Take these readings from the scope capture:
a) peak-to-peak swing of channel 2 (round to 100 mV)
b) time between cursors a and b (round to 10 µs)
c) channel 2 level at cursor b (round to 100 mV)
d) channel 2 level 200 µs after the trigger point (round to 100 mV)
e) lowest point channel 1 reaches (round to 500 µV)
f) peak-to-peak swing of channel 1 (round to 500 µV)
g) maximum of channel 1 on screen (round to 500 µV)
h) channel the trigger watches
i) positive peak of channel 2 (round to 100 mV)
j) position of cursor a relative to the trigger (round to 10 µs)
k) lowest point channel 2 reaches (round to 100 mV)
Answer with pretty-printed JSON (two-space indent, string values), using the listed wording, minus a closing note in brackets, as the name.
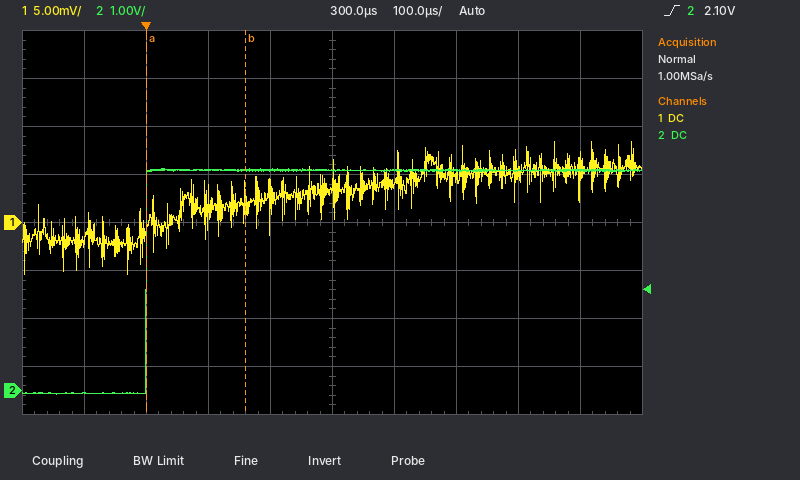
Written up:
{
  "peak-to-peak swing of channel 2": "4.7 V",
  "time between cursors a and b": "160 µs",
  "channel 2 level at cursor b": "4.6 V",
  "channel 2 level 200 µs after the trigger point": "4.6 V",
  "lowest point channel 1 reaches": "-5.5 mV",
  "peak-to-peak swing of channel 1": "14.0 mV",
  "maximum of channel 1 on screen": "8.5 mV",
  "channel the trigger watches": "channel 2",
  "positive peak of channel 2": "4.6 V",
  "position of cursor a relative to the trigger": "0 µs",
  "lowest point channel 2 reaches": "-100 mV"
}
